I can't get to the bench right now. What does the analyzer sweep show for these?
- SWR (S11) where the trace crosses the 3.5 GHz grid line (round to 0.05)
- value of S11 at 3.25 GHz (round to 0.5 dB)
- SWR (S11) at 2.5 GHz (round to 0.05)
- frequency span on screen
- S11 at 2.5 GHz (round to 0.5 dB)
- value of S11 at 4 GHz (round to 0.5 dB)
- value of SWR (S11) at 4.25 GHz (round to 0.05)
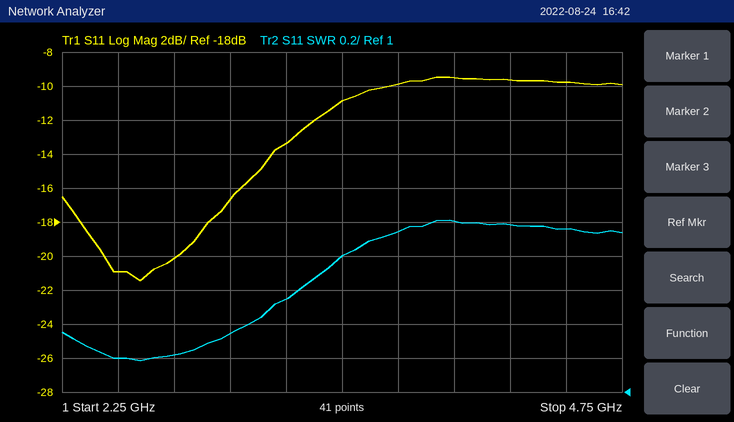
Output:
1.80
-13.5 dB
1.20
2.5 GHz
-21.0 dB
-9.5 dB
2.00
